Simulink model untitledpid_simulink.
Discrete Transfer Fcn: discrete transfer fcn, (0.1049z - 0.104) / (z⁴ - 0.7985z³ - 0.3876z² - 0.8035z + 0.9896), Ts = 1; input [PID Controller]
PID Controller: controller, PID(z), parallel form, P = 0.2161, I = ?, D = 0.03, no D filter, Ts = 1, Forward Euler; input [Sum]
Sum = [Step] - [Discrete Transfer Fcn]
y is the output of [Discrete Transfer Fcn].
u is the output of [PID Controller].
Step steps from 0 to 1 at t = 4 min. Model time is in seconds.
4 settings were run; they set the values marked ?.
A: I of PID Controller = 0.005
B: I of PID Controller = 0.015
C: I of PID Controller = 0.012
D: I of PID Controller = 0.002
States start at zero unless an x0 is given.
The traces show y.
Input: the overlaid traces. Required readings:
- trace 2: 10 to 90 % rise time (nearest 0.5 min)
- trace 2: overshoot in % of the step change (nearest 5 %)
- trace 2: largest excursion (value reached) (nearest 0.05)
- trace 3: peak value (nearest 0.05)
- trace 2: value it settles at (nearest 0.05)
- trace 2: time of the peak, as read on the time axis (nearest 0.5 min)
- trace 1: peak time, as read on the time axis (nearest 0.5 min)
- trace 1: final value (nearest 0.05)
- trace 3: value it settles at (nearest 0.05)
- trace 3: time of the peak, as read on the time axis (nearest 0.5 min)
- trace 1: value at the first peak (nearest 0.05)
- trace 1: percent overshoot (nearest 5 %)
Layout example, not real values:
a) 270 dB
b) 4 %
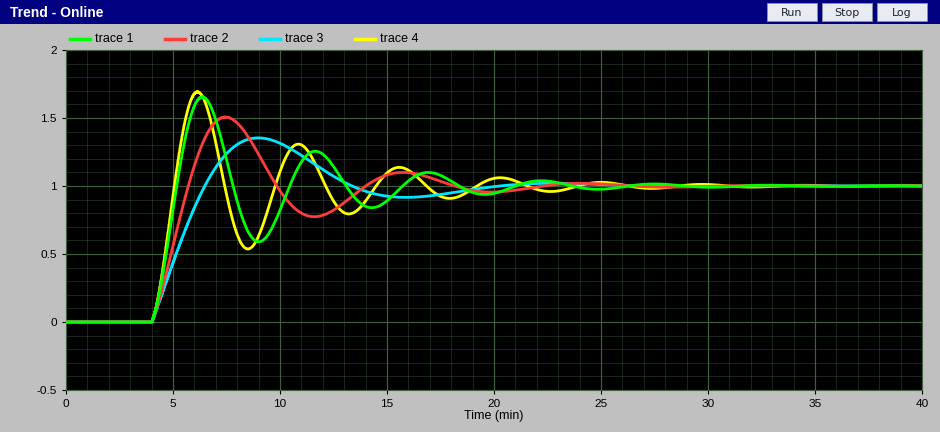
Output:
a) 1.5 min
b) 50 %
c) 1.50
d) 1.35
e) 1.00
f) 7.5 min
g) 6.5 min
h) 1.00
i) 1.00
j) 9.0 min
k) 1.65
l) 65 %
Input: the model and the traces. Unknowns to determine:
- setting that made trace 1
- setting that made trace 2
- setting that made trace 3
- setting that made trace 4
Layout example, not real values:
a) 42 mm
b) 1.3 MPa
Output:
a) C
b) A
c) D
d) B
